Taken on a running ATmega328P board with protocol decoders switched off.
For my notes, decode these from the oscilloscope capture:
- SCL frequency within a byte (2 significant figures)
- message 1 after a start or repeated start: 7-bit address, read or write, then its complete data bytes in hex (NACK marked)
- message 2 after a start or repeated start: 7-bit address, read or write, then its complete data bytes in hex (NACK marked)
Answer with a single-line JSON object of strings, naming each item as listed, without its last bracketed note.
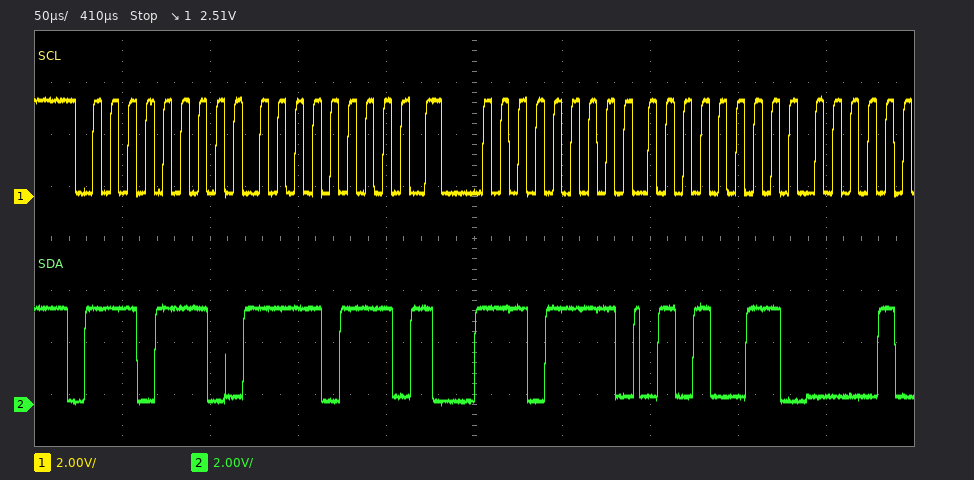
{"SCL frequency within a byte": "100 kHz", "message 1 after a start or repeated start: 7-bit address, read or write, then its complete data bytes in hex": "0x77 write: F7", "message 2 after a start or repeated start: 7-bit address, read or write, then its complete data bytes in hex": "0x77 read: 53"}
